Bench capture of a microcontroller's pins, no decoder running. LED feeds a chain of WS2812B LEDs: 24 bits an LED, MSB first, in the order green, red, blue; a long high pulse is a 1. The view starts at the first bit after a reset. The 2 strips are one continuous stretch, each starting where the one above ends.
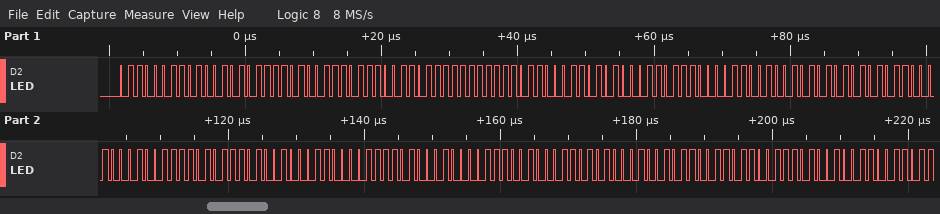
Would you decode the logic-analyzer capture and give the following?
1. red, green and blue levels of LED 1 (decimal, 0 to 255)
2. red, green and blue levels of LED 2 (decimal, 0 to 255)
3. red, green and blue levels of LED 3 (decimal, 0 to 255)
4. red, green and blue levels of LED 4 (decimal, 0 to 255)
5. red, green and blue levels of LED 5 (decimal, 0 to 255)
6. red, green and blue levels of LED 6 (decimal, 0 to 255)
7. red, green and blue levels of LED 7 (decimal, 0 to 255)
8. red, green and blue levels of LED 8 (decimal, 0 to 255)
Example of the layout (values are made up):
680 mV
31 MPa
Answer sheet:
74, 99, 244
111, 238, 254
163, 198, 112
85, 201, 88
235, 137, 164
232, 97, 135
81, 35, 44
210, 217, 102
